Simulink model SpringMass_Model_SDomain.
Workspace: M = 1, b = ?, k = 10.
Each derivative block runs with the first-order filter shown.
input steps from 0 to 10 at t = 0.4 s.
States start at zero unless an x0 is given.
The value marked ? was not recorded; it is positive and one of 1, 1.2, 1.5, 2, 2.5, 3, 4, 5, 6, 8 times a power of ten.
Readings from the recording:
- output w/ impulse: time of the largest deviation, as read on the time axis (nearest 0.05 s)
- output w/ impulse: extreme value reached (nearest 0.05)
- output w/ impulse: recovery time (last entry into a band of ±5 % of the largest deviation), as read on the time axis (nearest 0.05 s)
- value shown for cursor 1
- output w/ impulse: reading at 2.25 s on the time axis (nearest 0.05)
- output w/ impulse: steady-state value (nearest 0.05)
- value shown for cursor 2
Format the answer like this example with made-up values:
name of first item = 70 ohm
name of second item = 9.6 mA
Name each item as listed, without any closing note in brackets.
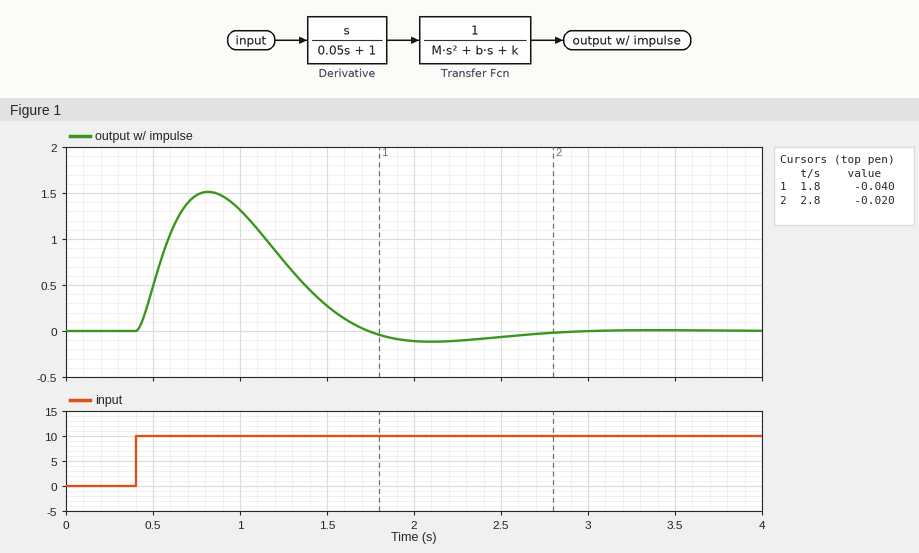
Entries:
output w/ impulse: time of the largest deviation, as read on the time axis = 0.80 s
output w/ impulse: extreme value reached = 1.50
output w/ impulse: recovery time (last entry into a band of ±5 % of the largest deviation), as read on the time axis = 2.45 s
value shown for cursor 1 = -0.040
output w/ impulse: reading at 2.25 s on the time axis = -0.10
output w/ impulse: steady-state value = 0.00
value shown for cursor 2 = -0.020
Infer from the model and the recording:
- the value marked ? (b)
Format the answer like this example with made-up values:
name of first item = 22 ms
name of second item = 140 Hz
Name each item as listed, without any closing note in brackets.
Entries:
the value marked ? = 4
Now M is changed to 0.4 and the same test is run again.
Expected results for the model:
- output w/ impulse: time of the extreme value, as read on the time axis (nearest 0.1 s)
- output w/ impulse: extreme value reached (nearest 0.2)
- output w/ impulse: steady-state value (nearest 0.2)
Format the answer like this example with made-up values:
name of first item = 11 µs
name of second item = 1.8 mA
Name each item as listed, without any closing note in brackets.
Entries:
output w/ impulse: time of the extreme value, as read on the time axis = 0.7 s
output w/ impulse: extreme value reached = 1.8
output w/ impulse: steady-state value = 0.0
